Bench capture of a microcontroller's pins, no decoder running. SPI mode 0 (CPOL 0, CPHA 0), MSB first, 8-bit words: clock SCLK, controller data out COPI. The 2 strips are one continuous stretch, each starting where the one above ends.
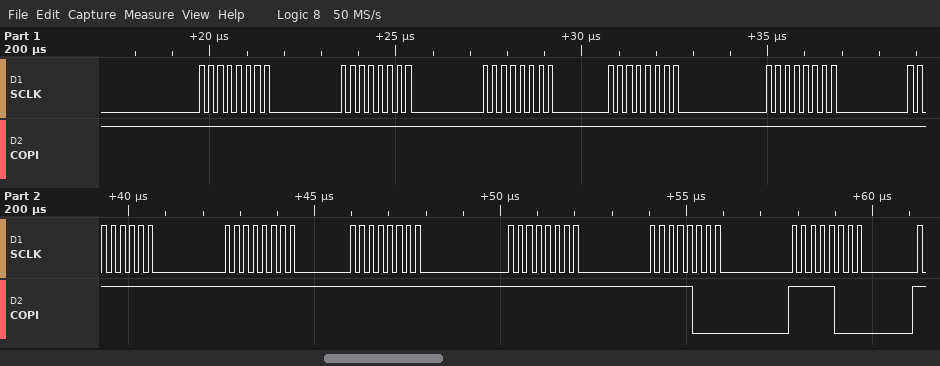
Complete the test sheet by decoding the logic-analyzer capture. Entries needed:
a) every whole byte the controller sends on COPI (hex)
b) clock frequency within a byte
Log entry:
FF FF FF FF FF FF FF FF FF F8 F8
4 MHz
